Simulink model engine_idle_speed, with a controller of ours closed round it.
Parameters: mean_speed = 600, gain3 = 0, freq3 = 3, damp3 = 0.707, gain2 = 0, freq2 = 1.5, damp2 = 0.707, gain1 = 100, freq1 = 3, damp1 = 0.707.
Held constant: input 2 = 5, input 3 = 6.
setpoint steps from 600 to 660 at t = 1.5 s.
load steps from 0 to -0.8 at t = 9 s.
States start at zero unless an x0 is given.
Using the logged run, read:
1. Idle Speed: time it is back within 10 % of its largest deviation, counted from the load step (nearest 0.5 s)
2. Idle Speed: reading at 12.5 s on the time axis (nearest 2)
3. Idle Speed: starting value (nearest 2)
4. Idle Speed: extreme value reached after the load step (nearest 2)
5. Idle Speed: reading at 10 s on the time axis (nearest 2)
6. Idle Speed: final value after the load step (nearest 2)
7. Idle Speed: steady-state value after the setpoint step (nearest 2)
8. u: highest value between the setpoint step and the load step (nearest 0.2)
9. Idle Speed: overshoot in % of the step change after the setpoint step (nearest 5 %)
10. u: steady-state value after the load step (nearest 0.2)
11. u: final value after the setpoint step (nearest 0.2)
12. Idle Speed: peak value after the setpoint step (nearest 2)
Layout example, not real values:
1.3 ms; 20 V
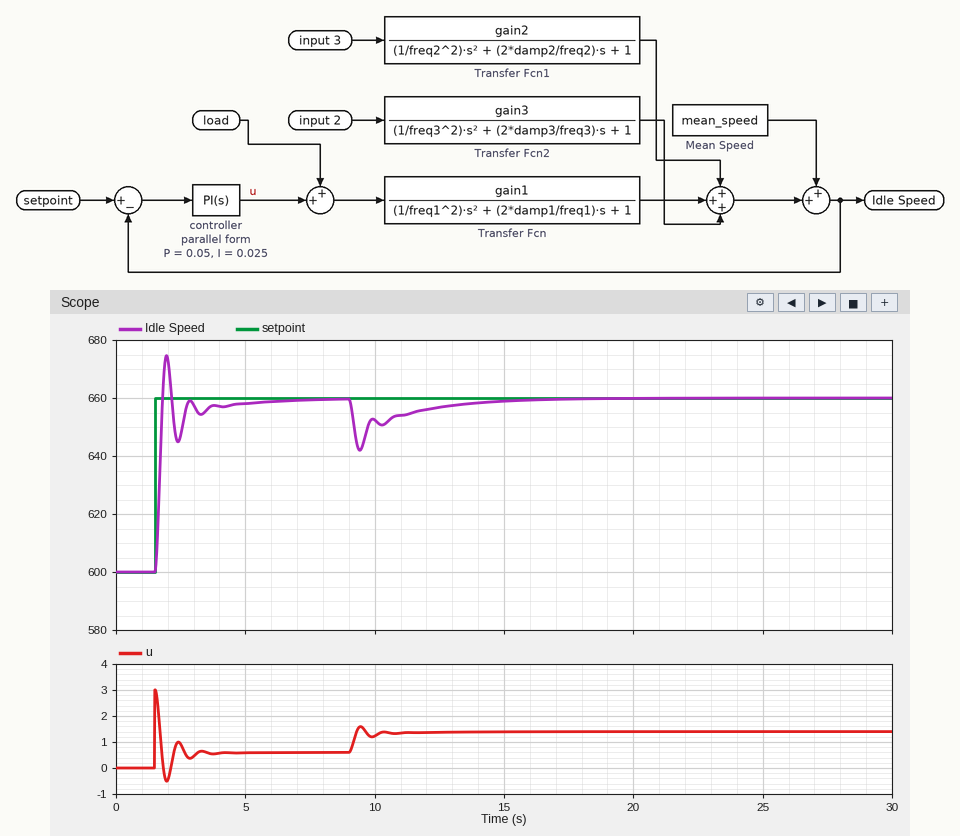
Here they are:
5.0 s; 656; 600; 642; 652; 660; 660; 3.0; 25 %; 1.4; 0.6; 674
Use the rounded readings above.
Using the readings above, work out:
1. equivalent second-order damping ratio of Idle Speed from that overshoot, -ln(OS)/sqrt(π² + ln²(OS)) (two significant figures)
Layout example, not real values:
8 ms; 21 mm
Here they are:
0.40
